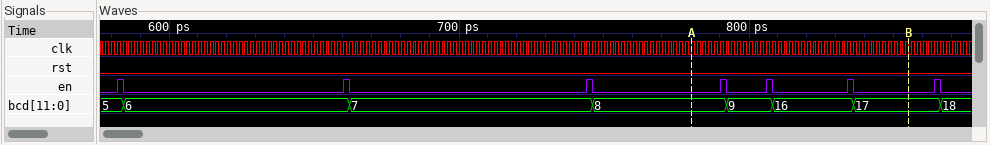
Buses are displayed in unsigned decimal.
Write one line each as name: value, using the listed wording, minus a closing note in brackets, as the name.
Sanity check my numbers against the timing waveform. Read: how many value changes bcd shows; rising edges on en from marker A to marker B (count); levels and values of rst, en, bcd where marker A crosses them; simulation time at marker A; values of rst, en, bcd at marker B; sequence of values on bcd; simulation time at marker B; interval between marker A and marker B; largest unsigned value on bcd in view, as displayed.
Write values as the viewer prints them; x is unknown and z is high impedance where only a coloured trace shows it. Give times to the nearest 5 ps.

how many value changes bcd shows: 7
rising edges on en from marker A to marker B: 3
levels and values of rst, en, bcd where marker A crosses them: rst=0, en=0, bcd=8
simulation time at marker A: 780 ps
values of rst, en, bcd at marker B: rst=0, en=0, bcd=17
sequence of values on bcd: 5, 6, 7, 8, 9, 16, 17, 18
simulation time at marker B: 855 ps
interval between marker A and marker B: 75 ps
largest unsigned value on bcd in view, as displayed: 18
